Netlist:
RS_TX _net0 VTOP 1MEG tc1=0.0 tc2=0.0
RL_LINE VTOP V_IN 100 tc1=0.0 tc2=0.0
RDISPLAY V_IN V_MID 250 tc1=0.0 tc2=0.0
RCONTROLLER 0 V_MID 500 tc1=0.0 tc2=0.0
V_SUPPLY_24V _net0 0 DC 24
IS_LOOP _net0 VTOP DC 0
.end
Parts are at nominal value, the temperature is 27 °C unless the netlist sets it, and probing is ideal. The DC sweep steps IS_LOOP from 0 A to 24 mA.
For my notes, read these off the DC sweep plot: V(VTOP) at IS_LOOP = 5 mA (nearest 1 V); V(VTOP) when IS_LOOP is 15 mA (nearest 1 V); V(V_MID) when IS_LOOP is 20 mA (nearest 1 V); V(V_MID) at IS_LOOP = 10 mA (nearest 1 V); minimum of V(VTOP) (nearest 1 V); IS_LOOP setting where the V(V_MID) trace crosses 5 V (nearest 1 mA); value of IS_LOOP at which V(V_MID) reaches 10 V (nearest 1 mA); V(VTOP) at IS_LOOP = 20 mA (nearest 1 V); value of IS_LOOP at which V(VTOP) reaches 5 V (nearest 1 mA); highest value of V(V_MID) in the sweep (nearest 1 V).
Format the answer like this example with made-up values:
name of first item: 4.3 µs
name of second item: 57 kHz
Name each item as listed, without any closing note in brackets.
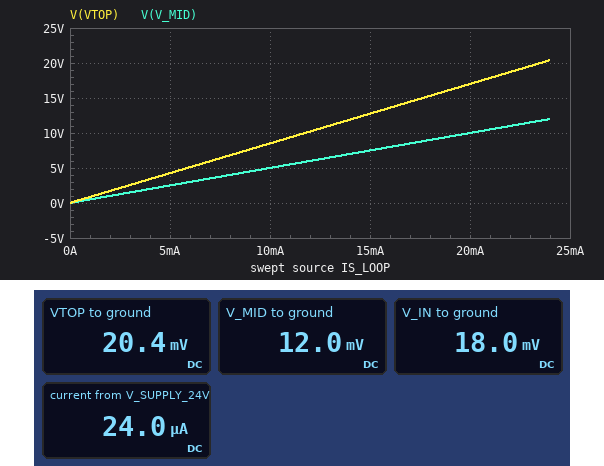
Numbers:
V(VTOP) at IS_LOOP = 5 mA: 4 V
V(VTOP) when IS_LOOP is 15 mA: 13 V
V(V_MID) when IS_LOOP is 20 mA: 10 V
V(V_MID) at IS_LOOP = 10 mA: 5 V
minimum of V(VTOP): 0 V
IS_LOOP setting where the V(V_MID) trace crosses 5 V: 10 mA
value of IS_LOOP at which V(V_MID) reaches 10 V: 20 mA
V(VTOP) at IS_LOOP = 20 mA: 17 V
value of IS_LOOP at which V(VTOP) reaches 5 V: 6 mA
highest value of V(V_MID) in the sweep: 12 V
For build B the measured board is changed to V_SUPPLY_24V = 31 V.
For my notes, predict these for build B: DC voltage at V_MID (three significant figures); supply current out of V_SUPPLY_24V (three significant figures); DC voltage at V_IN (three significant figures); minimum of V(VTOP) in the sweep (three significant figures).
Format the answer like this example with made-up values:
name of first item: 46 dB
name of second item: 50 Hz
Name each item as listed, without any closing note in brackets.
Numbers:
DC voltage at V_MID: 15.5 mV
supply current out of V_SUPPLY_24V: 31.0 µA
DC voltage at V_IN: 23.2 mV
minimum of V(VTOP) in the sweep: 26.3 mV
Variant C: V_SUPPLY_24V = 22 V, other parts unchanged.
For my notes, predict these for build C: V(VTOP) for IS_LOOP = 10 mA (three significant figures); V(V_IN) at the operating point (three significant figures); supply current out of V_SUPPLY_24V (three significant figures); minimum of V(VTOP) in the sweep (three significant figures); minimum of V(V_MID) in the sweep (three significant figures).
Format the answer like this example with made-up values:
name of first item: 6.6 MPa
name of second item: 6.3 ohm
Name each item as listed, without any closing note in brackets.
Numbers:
V(VTOP) for IS_LOOP = 10 mA: 8.51 V
V(V_IN) at the operating point: 16.5 mV
supply current out of V_SUPPLY_24V: 22.0 µA
minimum of V(VTOP) in the sweep: 18.7 mV
minimum of V(V_MID) in the sweep: 11.0 mV
